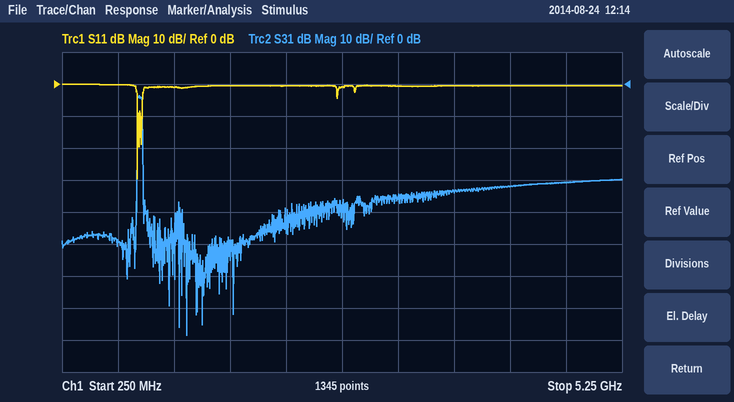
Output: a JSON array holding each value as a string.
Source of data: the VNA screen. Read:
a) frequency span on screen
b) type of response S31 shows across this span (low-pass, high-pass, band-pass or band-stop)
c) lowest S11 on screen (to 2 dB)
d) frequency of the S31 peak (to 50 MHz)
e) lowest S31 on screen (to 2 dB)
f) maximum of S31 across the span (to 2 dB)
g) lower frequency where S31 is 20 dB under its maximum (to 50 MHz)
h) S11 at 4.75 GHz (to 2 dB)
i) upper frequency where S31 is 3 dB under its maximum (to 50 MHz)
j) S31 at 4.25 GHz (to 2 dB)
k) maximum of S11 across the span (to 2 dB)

["5 GHz", "band-pass", "-30 dB", "950 MHz", "-78 dB", "-4 dB", "900 MHz", "0 dB", "950 MHz", "-32 dB", "0 dB"]
